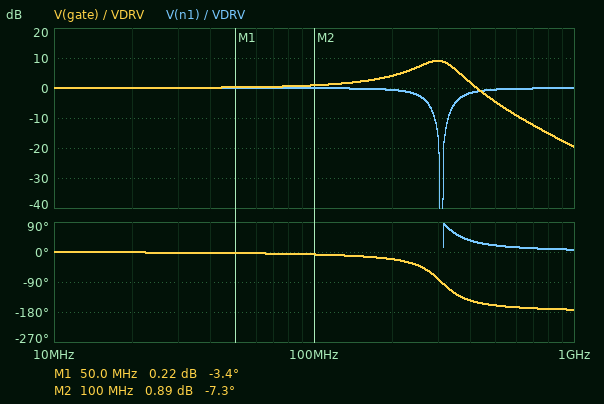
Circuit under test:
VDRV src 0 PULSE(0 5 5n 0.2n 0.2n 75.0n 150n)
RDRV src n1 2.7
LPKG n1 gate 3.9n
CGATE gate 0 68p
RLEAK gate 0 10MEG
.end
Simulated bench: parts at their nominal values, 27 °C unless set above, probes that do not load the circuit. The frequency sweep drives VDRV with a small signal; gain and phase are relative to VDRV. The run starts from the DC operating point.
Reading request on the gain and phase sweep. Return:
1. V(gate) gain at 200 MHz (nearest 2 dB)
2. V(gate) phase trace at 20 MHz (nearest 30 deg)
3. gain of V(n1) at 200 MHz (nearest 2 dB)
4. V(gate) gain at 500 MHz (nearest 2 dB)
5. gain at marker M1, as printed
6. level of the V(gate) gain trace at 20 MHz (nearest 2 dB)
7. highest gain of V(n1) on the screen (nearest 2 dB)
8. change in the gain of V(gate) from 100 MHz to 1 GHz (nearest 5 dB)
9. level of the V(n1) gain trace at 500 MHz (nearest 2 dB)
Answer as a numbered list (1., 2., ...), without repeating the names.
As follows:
1. 4 dB
2. 0 deg
3. 0 dB
4. -4 dB
5. 0.22 dB
6. 0 dB
7. 0 dB
8. -20 dB
9. 0 dB
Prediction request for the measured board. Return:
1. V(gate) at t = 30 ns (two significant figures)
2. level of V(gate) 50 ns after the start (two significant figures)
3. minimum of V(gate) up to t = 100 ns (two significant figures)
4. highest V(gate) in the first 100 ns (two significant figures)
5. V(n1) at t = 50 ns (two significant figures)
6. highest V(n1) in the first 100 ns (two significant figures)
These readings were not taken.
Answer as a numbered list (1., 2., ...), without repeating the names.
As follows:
1. 5.0 V
2. 5.0 V
3. -2.8 V
4. 7.8 V
5. 5.0 V
6. 5.8 V
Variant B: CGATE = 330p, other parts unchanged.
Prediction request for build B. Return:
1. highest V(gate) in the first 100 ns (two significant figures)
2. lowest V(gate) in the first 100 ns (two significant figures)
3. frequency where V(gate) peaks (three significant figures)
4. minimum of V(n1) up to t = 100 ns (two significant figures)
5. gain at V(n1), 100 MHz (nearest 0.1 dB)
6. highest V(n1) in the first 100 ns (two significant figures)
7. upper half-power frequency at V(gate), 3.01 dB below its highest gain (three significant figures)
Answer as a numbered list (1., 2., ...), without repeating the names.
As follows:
1. 6.3 V
2. -1.3 V
3. 117 MHz
4. -620 mV
5. -3.6 dB
6. 5.6 V
7. 167 MHz
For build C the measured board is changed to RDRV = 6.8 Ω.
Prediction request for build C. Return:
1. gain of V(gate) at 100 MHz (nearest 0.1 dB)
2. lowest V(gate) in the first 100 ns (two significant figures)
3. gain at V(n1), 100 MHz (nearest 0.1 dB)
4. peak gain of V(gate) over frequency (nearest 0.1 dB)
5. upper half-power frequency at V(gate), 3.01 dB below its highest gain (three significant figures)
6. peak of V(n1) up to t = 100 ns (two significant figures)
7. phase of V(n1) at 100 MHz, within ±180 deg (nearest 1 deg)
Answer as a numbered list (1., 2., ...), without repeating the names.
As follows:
1. 0.5 dB
2. -1.0 V
3. -0.4 dB
4. 1.9 dB
5. 366 MHz
6. 5.5 V
7. -18 deg
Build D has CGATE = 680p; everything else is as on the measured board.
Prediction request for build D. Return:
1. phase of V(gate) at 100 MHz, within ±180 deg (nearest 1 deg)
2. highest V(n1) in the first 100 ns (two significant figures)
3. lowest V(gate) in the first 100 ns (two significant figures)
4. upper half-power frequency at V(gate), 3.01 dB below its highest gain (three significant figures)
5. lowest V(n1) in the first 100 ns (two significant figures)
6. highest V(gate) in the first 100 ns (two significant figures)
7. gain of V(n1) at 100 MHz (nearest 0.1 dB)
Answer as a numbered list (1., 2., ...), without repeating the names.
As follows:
1. -92 deg
2. 5.3 V
3. -590 mV
4. 111 MHz
5. -340 mV
6. 5.6 V
7. -27.8 dB
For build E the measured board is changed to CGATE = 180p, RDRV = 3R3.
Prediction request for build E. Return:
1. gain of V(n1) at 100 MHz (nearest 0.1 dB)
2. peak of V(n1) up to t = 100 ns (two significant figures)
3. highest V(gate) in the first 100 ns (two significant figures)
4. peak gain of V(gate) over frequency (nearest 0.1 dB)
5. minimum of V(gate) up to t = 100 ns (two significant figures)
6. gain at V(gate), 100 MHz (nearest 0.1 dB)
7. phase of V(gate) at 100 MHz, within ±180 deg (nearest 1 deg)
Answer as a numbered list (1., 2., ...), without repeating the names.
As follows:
1. -1.0 dB
2. 5.7 V
3. 6.5 V
4. 3.6 dB
5. -1.5 V
6. 1.8 dB
7. -27 deg
